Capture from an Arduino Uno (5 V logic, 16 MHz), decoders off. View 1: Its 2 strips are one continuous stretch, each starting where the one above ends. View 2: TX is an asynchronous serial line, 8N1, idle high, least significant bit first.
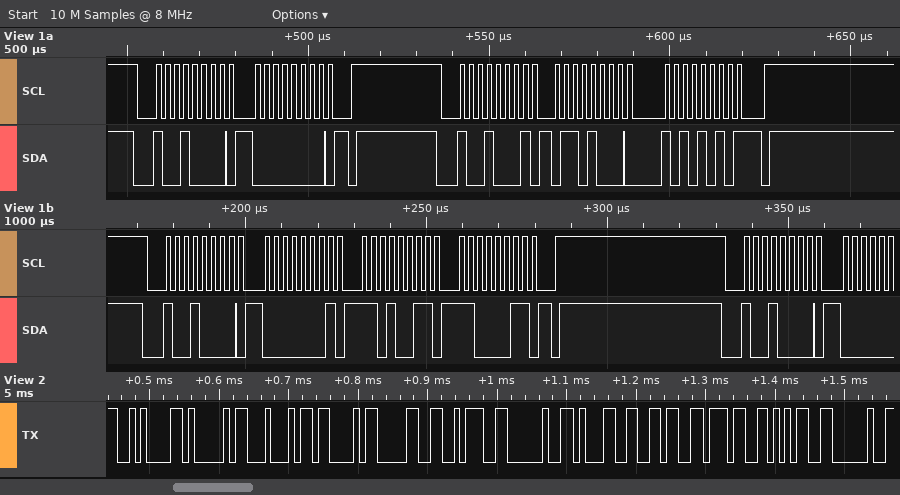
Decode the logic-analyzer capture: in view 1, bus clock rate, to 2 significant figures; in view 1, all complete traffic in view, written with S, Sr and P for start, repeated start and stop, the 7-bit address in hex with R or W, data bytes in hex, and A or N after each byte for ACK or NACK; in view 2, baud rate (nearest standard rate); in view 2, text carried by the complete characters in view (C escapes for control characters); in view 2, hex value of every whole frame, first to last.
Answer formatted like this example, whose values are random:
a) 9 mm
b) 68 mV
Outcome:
a) 400 kHz
b) S 48W A 00 A P S 48R A 68 A AA N P S 48W A 01 A D3 A C3 A P S 48W A
c) 115200 baud
d) "\nADC0: 1675 "
e) 0A 41 44 43 30 3A 20 31 36 37 35 20
